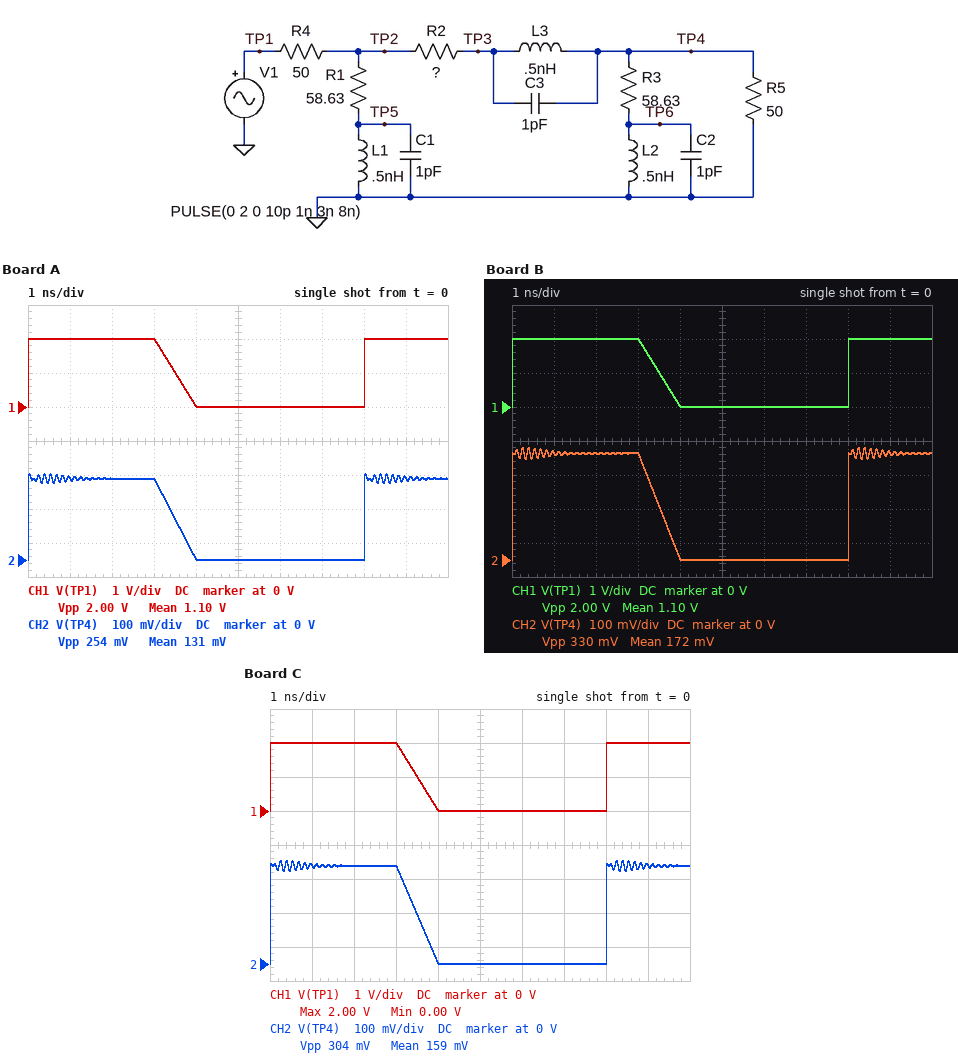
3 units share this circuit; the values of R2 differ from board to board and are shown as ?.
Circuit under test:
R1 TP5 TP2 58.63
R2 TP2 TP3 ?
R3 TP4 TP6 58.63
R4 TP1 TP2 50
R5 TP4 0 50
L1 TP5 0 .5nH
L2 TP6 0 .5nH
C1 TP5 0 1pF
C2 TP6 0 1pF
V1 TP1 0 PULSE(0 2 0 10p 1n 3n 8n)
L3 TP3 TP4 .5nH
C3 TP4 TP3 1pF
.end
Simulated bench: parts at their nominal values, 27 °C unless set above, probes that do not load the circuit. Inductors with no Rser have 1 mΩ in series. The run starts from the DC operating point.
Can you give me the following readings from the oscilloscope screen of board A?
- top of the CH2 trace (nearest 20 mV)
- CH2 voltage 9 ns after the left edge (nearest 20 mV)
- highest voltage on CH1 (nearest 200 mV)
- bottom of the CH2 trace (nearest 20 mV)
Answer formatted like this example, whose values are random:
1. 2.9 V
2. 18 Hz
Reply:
1. 260 mV
2. 240 mV
3. 2.0 V
4. 0 V
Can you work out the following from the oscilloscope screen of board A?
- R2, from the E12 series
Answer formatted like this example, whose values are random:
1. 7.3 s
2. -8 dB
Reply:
1. 68 Ω
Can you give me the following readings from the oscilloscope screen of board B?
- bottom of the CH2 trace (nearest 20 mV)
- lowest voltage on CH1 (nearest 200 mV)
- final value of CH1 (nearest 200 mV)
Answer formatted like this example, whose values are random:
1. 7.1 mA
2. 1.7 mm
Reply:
1. 0 V
2. 0 V
3. 2.0 V
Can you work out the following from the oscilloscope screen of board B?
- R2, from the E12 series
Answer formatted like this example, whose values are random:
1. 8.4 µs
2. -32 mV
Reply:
1. 39 Ω
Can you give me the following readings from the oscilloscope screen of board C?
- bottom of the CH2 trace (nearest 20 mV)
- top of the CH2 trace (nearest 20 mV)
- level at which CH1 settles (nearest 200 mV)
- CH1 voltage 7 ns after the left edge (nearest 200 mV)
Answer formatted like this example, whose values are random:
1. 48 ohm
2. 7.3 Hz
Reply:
1. 0 V
2. 300 mV
3. 2.0 V
4. 0 V
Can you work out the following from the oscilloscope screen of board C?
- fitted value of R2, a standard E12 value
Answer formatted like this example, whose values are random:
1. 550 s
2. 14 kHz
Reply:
1. 47 Ω
